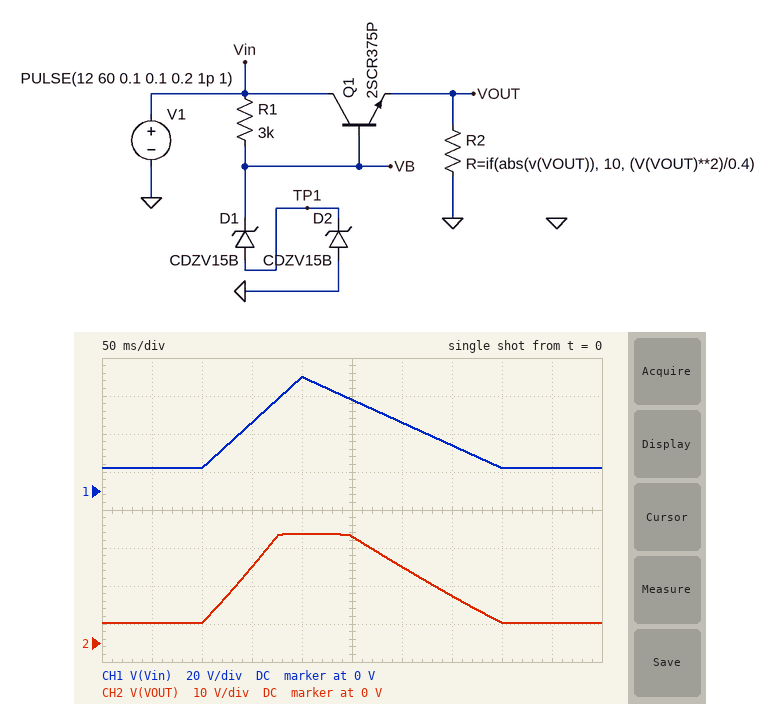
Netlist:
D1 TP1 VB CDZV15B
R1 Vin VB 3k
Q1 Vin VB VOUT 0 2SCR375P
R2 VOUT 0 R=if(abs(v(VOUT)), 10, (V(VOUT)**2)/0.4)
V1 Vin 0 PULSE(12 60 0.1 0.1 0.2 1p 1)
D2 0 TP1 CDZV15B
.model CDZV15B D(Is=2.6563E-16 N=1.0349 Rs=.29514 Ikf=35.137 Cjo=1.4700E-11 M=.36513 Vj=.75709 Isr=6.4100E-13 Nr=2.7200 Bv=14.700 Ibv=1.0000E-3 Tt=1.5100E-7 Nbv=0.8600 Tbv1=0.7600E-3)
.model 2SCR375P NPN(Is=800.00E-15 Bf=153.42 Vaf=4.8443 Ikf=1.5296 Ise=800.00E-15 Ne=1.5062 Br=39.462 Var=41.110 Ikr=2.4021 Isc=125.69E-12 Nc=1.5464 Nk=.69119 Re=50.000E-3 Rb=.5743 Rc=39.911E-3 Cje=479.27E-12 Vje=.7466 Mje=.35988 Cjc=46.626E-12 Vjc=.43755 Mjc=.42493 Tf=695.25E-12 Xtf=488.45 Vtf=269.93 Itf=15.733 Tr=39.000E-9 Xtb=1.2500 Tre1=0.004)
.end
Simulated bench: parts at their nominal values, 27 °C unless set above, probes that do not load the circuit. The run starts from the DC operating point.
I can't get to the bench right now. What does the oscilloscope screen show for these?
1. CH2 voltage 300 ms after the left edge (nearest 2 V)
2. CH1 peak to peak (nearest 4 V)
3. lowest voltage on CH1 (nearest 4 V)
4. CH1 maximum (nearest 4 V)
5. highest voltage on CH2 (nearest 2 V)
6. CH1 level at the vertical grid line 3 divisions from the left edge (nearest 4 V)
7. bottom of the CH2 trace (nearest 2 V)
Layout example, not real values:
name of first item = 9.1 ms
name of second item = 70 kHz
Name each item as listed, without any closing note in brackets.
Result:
CH2 voltage 300 ms after the left edge = 20 V
CH1 peak to peak = 48 V
lowest voltage on CH1 = 12 V
CH1 maximum = 60 V
highest voltage on CH2 = 28 V
CH1 level at the vertical grid line 3 divisions from the left edge = 36 V
bottom of the CH2 trace = 6 V
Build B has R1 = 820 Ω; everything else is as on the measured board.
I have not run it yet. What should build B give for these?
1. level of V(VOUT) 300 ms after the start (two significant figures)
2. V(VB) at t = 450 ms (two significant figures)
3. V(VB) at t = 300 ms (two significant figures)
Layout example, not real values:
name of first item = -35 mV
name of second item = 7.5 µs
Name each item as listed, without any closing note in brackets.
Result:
level of V(VOUT) 300 ms after the start = 25 V
V(VB) at t = 450 ms = 8.4 V
V(VB) at t = 300 ms = 26 V
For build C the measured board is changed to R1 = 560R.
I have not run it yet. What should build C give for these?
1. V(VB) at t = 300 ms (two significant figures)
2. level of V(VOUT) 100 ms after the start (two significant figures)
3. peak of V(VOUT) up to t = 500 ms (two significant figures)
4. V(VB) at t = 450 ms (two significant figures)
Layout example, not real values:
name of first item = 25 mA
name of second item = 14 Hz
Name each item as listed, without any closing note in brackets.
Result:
V(VB) at t = 300 ms = 27 V
level of V(VOUT) 100 ms after the start = 8.2 V
peak of V(VOUT) up to t = 500 ms = 29 V
V(VB) at t = 450 ms = 9.0 V
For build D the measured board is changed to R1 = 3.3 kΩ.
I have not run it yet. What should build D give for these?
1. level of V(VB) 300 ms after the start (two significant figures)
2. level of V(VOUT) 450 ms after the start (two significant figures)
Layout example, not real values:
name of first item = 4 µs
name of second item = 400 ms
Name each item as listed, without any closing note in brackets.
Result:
level of V(VB) 300 ms after the start = 20 V
level of V(VOUT) 450 ms after the start = 5.1 V
